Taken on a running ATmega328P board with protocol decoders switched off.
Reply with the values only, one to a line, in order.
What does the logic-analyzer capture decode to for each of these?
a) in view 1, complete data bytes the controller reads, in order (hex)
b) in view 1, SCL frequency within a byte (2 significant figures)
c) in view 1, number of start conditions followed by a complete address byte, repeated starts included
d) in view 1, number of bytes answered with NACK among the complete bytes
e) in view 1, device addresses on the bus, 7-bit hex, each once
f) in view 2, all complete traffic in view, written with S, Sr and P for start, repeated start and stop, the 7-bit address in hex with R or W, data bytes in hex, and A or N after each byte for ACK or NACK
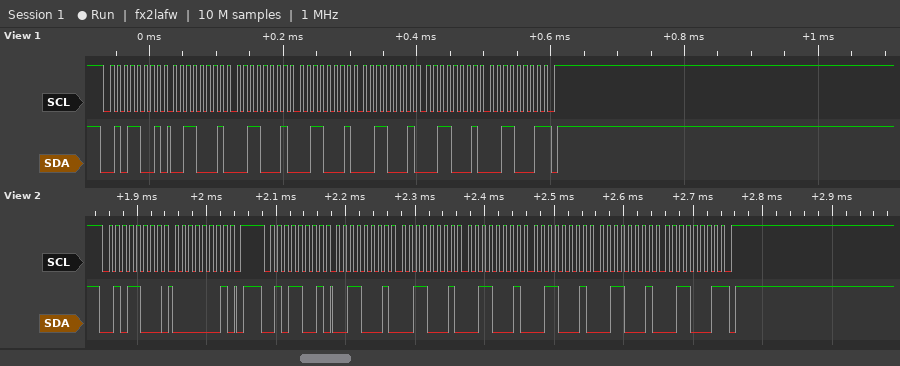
31 31 31 31 31 31
100 kHz
1
1
0x2C
S 2CW A 01 A P S 2CR A 31 A 31 A 31 A 31 A 31 A 31 N P
